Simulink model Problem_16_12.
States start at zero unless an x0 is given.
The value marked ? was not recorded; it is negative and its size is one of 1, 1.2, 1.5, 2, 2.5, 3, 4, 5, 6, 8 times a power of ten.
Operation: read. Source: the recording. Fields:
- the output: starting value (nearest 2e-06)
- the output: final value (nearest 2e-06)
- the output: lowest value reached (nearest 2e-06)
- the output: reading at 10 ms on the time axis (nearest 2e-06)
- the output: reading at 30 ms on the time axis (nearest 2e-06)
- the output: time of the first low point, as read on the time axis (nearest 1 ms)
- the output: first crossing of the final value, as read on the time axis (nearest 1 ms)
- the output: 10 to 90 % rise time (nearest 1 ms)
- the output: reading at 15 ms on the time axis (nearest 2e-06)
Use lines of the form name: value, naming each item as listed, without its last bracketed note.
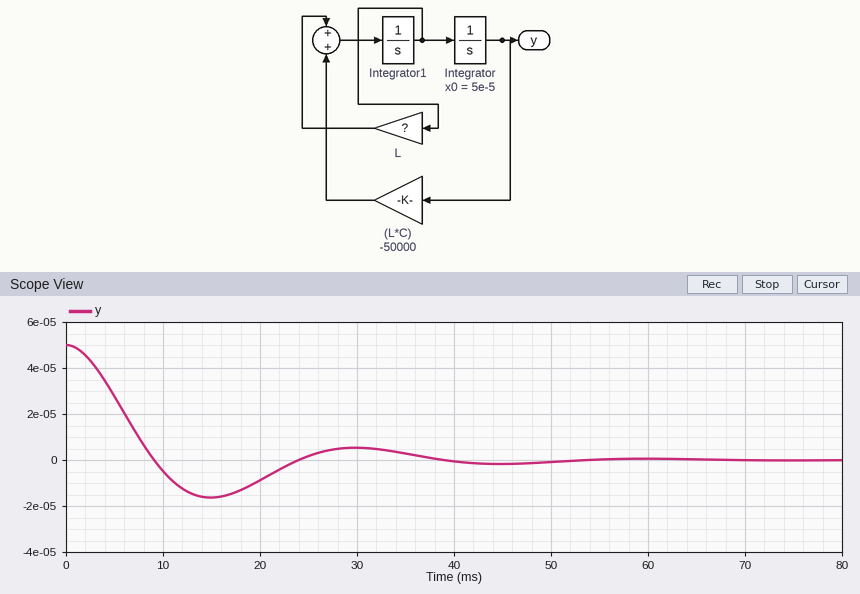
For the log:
the output: starting value: 0.000050
the output: final value: 0.000000
the output: lowest value reached: -0.000016
the output: reading at 10 ms on the time axis: -0.000004
the output: reading at 30 ms on the time axis: 0.000006
the output: time of the first low point, as read on the time axis: 15 ms
the output: first crossing of the final value, as read on the time axis: 9 ms
the output: 10 to 90 % rise time: 6 ms
the output: reading at 15 ms on the time axis: -0.000016
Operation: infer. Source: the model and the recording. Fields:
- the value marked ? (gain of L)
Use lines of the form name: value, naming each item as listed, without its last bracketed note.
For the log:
the value marked ?: -150
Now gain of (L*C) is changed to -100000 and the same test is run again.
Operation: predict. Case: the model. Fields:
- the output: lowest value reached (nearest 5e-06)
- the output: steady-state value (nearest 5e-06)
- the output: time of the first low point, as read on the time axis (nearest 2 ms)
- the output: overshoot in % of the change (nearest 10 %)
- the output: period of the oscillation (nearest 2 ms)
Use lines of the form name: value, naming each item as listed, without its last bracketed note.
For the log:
the output: lowest value reached: -0.000025
the output: steady-state value: 0.000000
the output: time of the first low point, as read on the time axis: 10 ms
the output: overshoot in % of the change: 50 %
the output: period of the oscillation: 20 ms
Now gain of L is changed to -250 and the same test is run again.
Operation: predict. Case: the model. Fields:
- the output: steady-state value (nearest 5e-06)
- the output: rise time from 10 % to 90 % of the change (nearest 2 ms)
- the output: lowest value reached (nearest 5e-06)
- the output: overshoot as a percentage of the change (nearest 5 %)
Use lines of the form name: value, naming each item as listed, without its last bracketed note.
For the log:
the output: steady-state value: 0.000000
the output: rise time from 10 % to 90 % of the change: 8 ms
the output: lowest value reached: -0.000005
the output: overshoot as a percentage of the change: 10 %
